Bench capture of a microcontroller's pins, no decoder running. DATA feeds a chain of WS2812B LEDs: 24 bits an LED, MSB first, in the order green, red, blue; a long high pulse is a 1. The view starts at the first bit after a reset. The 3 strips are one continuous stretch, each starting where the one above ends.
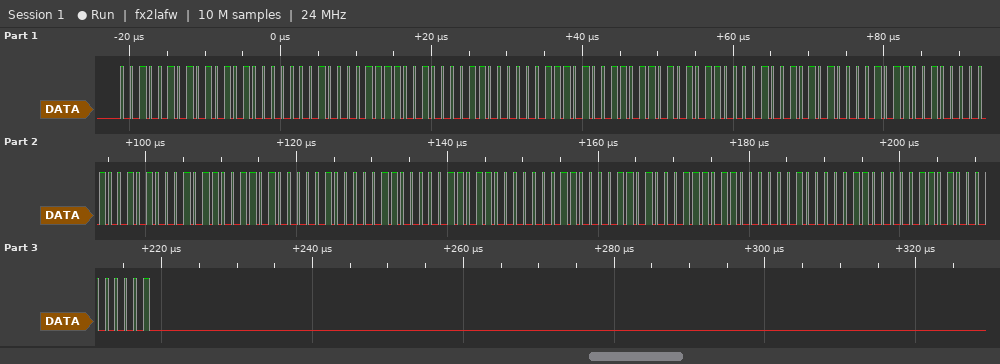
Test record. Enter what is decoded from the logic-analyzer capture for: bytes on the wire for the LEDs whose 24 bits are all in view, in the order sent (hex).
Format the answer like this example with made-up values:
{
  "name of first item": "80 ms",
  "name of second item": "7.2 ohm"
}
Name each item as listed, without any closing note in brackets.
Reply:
{
  "bytes on the wire for the LEDs whose 24 bits are all in view, in the order sent": "25 54 04 3C 86 07 4D AB 09 50 B2 09 45 9A 08 30 6C 06 1A 3B 02 0C 1A 01"
}
